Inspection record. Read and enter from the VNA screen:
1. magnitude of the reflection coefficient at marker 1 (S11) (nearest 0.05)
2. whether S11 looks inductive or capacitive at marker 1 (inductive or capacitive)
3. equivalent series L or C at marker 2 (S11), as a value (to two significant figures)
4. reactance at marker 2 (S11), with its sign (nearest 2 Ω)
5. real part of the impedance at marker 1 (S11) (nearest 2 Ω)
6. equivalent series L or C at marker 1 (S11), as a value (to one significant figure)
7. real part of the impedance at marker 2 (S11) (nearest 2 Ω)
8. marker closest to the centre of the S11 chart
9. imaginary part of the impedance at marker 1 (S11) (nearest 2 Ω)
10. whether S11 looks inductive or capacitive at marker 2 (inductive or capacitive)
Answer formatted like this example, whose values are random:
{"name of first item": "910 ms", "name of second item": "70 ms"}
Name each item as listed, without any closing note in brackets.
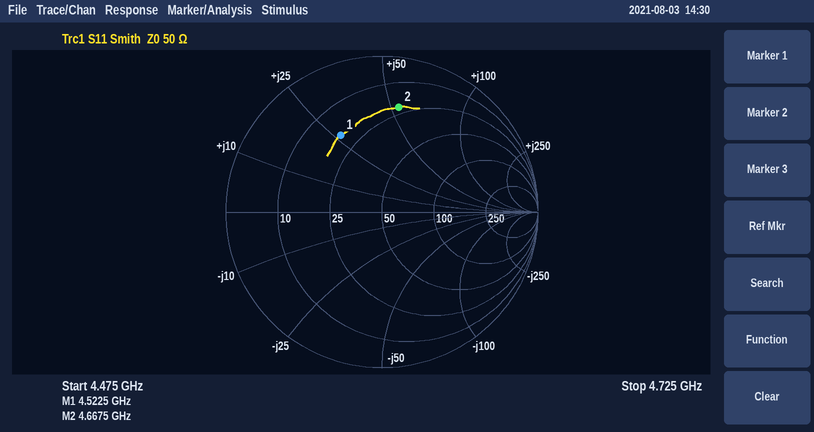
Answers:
{"magnitude of the reflection coefficient at marker 1 (S11)": "0.55", "whether S11 looks inductive or capacitive at marker 1": "inductive", "equivalent series L or C at marker 2 (S11), as a value": "1.8 nH", "reactance at marker 2 (S11), with its sign": "+54 Ω", "real part of the impedance at marker 1 (S11)": "18 Ω", "equivalent series L or C at marker 1 (S11), as a value": "900 pH", "real part of the impedance at marker 2 (S11)": "22 Ω", "marker closest to the centre of the S11 chart": "marker 1", "imaginary part of the impedance at marker 1 (S11)": "+26 Ω", "whether S11 looks inductive or capacitive at marker 2": "inductive"}
